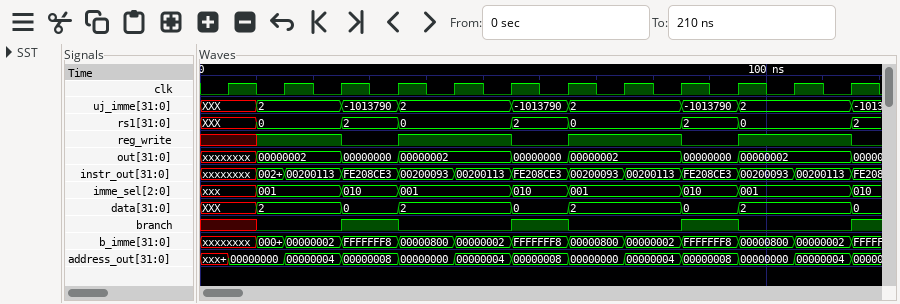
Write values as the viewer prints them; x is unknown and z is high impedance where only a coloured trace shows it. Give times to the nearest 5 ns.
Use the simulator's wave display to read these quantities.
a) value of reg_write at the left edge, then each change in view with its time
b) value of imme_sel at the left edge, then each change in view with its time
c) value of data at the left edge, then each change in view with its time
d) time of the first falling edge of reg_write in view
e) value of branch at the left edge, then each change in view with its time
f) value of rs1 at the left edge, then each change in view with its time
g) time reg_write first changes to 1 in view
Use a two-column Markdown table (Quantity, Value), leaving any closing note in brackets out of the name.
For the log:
| Quantity | Value |
|---|---|
| value of reg_write at the left edge, then each change in view with its time | x, 1 at 10 ns, 0 at 25 ns, 1 at 35 ns, 0 at 55 ns, 1 at 65 ns, 0 at 85 ns, 1 at 95 ns, 0 at 115 ns |
| value of imme_sel at the left edge, then each change in view with its time | xxx, 001 at 10 ns, 010 at 25 ns, 001 at 35 ns, 010 at 55 ns, 001 at 65 ns, 010 at 85 ns, 001 at 95 ns, 010 at 115 ns |
| value of data at the left edge, then each change in view with its time | XXX, 2 at 10 ns, 0 at 25 ns, 2 at 35 ns, 0 at 55 ns, 2 at 65 ns, 0 at 85 ns, 2 at 95 ns, 0 at 115 ns |
| time of the first falling edge of reg_write in view | 25 ns |
| value of branch at the left edge, then each change in view with its time | x, 0 at 10 ns, 1 at 25 ns, 0 at 35 ns, 1 at 55 ns, 0 at 65 ns, 1 at 85 ns, 0 at 95 ns, 1 at 115 ns |
| value of rs1 at the left edge, then each change in view with its time | XXX, 0 at 10 ns, 2 at 25 ns, 0 at 35 ns, 2 at 55 ns, 0 at 65 ns, 2 at 85 ns, 0 at 95 ns, 2 at 115 ns |
| time reg_write first changes to 1 in view | 10 ns |
